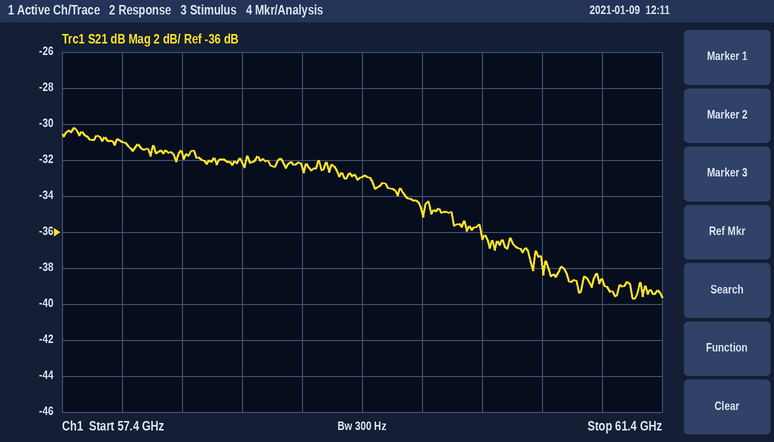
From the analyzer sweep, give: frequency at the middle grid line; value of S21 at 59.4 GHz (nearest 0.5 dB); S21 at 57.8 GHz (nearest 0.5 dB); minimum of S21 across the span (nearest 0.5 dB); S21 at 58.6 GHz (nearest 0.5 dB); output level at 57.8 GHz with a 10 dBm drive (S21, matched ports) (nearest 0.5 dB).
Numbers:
59.4 GHz
-33.0 dB
-31.0 dB
-39.5 dB
-32.0 dB
-21.0 dBm
